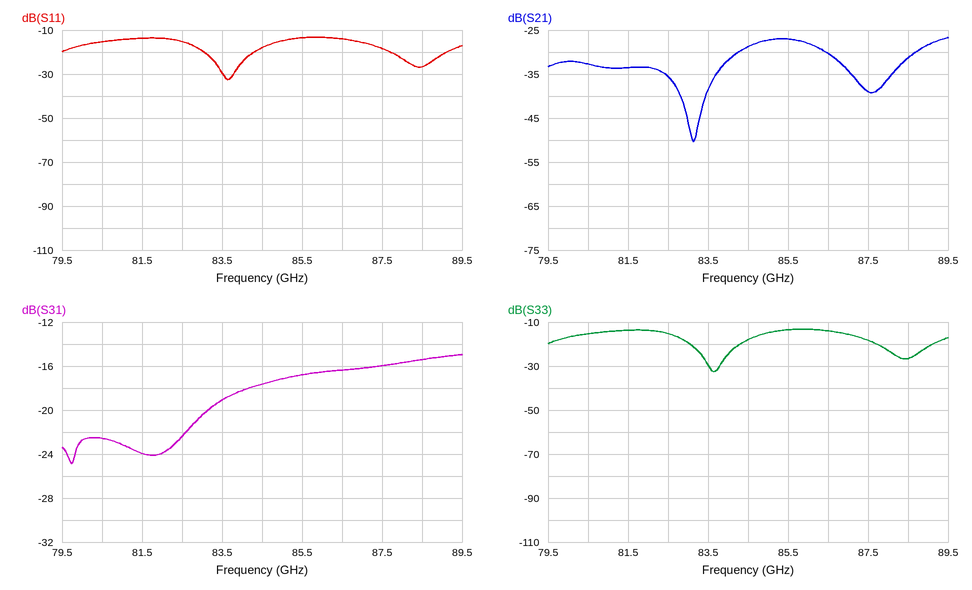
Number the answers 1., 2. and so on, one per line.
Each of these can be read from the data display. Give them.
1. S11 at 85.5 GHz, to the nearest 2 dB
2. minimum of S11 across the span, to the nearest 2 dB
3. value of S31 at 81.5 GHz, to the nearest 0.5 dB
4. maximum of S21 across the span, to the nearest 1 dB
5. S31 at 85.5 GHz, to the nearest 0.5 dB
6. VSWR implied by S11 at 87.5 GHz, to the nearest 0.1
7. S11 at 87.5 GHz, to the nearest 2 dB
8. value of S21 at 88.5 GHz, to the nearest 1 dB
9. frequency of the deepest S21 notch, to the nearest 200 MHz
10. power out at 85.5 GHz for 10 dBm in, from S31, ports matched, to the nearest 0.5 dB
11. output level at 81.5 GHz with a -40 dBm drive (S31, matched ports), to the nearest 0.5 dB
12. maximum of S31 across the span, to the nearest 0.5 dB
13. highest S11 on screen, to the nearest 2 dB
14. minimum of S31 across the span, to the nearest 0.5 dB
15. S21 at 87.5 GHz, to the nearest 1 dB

1. -14 dB
2. -32 dB
3. -24.0 dB
4. -27 dB
5. -17.0 dB
6. 1.3
7. -18 dB
8. -31 dB
9. 83.2 GHz
10. -7.0 dBm
11. -64.0 dBm
12. -15.0 dB
13. -14 dB
14. -25.0 dB
15. -39 dB
